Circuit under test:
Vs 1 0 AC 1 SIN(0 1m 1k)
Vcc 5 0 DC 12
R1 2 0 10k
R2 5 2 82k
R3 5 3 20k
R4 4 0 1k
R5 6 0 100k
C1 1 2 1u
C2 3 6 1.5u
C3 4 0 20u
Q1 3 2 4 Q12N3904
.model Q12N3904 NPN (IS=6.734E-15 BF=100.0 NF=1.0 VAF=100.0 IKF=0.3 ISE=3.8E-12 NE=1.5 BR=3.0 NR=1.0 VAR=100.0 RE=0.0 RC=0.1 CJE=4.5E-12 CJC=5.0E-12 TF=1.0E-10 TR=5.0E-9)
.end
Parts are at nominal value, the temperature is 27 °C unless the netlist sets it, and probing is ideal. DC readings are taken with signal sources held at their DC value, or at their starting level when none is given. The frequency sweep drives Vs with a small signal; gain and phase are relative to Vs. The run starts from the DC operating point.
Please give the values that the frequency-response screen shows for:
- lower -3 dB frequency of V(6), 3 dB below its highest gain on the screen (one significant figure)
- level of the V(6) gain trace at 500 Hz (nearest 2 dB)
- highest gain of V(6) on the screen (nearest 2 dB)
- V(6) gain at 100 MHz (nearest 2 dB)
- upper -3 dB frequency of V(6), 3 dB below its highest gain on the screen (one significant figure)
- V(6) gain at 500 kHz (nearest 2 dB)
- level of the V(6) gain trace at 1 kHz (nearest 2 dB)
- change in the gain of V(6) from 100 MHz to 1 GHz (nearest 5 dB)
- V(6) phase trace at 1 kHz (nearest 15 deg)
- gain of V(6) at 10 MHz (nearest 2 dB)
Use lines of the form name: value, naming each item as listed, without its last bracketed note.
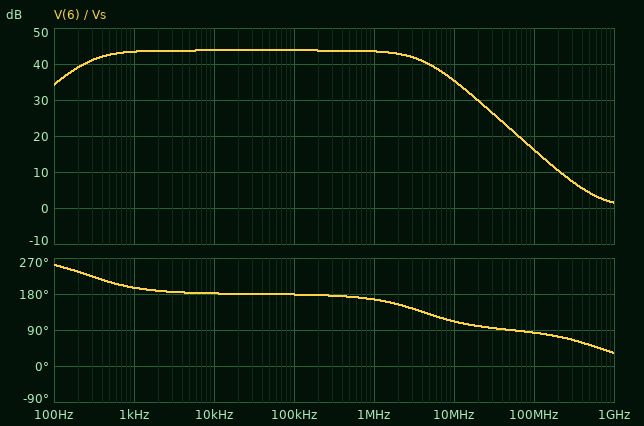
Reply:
lower -3 dB frequency of V(6), 3 dB below its highest gain on the screen: 300 Hz
level of the V(6) gain trace at 500 Hz: 42 dB
highest gain of V(6) on the screen: 44 dB
V(6) gain at 100 MHz: 16 dB
upper -3 dB frequency of V(6), 3 dB below its highest gain on the screen: 4 MHz
V(6) gain at 500 kHz: 44 dB
level of the V(6) gain trace at 1 kHz: 44 dB
change in the gain of V(6) from 100 MHz to 1 GHz: -15 dB
V(6) phase trace at 1 kHz: 195 deg
gain of V(6) at 10 MHz: 36 dB
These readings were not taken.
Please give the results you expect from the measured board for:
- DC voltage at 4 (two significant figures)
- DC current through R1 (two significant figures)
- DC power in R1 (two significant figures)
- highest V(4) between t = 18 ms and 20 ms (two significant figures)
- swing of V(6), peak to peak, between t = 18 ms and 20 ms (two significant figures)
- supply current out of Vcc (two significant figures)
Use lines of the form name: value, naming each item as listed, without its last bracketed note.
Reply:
DC voltage at 4: 290 mV
DC current through R1: 92 µA
DC power in R1: 85 µW
highest V(4) between t = 18 ms and 20 ms: 290 mV
swing of V(6), peak to peak, between t = 18 ms and 20 ms: 300 mV
supply current out of Vcc: 380 µA
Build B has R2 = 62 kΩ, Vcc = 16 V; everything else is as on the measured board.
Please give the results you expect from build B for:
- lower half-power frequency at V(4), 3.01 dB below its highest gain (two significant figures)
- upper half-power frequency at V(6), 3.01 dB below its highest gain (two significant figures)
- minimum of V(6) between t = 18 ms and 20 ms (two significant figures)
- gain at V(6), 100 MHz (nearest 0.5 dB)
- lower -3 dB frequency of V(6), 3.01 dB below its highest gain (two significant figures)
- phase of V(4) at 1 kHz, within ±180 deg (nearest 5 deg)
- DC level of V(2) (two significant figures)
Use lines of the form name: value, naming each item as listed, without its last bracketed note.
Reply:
lower half-power frequency at V(4), 3.01 dB below its highest gain: 11 Hz
upper half-power frequency at V(6), 3.01 dB below its highest gain: 2.6 MHz
minimum of V(6) between t = 18 ms and 20 ms: -340 mV
gain at V(6), 100 MHz: 20.5 dB
lower -3 dB frequency of V(6), 3.01 dB below its highest gain: 610 Hz
phase of V(4) at 1 kHz, within ±180 deg: -60 deg
DC level of V(2): 1.4 V
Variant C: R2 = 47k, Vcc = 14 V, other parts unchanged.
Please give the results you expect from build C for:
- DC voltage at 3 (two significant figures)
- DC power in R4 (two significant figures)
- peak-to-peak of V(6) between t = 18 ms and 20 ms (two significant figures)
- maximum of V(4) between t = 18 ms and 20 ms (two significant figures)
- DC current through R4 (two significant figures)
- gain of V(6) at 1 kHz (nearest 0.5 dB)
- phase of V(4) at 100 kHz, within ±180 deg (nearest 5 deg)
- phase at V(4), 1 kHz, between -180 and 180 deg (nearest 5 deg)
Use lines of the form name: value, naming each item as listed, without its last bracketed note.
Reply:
DC voltage at 3: 840 mV
DC power in R4: 610 µW
peak-to-peak of V(6) between t = 18 ms and 20 ms: 6.5 mV
maximum of V(4) between t = 18 ms and 20 ms: 780 mV
DC current through R4: 780 µA
gain of V(6) at 1 kHz: 10.0 dB
phase of V(4) at 100 kHz, within ±180 deg: -90 deg
phase at V(4), 1 kHz, between -180 and 180 deg: -30 deg
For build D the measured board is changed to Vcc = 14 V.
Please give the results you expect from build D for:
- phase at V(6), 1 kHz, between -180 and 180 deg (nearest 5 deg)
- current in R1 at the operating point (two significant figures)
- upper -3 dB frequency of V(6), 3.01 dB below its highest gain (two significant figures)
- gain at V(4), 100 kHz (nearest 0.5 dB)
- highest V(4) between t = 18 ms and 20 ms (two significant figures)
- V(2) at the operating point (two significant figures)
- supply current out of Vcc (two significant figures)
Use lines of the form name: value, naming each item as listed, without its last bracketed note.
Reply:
phase at V(6), 1 kHz, between -180 and 180 deg: -160 deg
current in R1 at the operating point: 100 µA
upper -3 dB frequency of V(6), 3.01 dB below its highest gain: 4.2 MHz
gain at V(4), 100 kHz: -59.0 dB
highest V(4) between t = 18 ms and 20 ms: 400 mV
V(2) at the operating point: 1.0 V
supply current out of Vcc: 510 µA
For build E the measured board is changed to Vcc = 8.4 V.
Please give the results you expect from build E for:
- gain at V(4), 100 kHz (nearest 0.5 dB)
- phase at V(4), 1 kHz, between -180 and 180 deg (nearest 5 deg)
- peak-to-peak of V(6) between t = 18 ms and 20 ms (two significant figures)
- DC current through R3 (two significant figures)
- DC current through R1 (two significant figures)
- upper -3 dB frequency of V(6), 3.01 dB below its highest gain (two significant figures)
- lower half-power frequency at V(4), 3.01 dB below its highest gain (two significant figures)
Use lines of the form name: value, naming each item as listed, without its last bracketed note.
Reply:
gain at V(4), 100 kHz: -69.5 dB
phase at V(4), 1 kHz, between -180 and 180 deg: -80 deg
peak-to-peak of V(6) between t = 18 ms and 20 ms: 120 mV
DC current through R3: 93 µA
DC current through R1: 72 µA
upper -3 dB frequency of V(6), 3.01 dB below its highest gain: 4.0 MHz
lower half-power frequency at V(4), 3.01 dB below its highest gain: 9.1 Hz
